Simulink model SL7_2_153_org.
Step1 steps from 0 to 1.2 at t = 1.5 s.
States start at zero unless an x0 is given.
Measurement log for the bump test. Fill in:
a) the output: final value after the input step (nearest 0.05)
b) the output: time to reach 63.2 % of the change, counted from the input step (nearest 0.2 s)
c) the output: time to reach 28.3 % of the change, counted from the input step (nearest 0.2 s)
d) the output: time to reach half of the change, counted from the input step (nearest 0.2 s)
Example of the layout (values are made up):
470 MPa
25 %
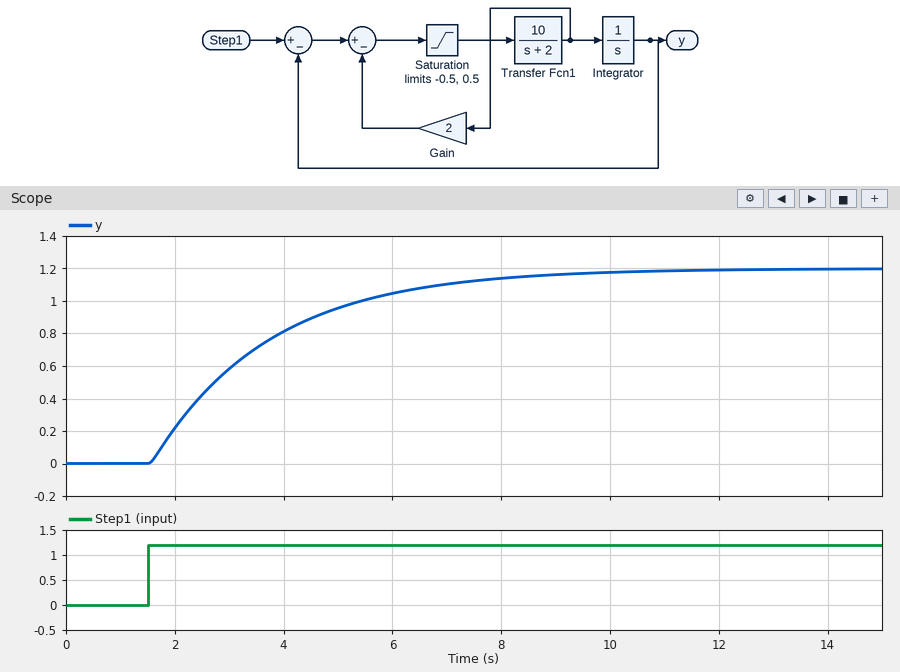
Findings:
1.20
2.2 s
0.8 s
1.6 s
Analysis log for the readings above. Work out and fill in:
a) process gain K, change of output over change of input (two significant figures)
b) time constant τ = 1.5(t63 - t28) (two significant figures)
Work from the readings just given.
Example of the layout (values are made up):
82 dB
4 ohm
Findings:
1.0
2.1 s
